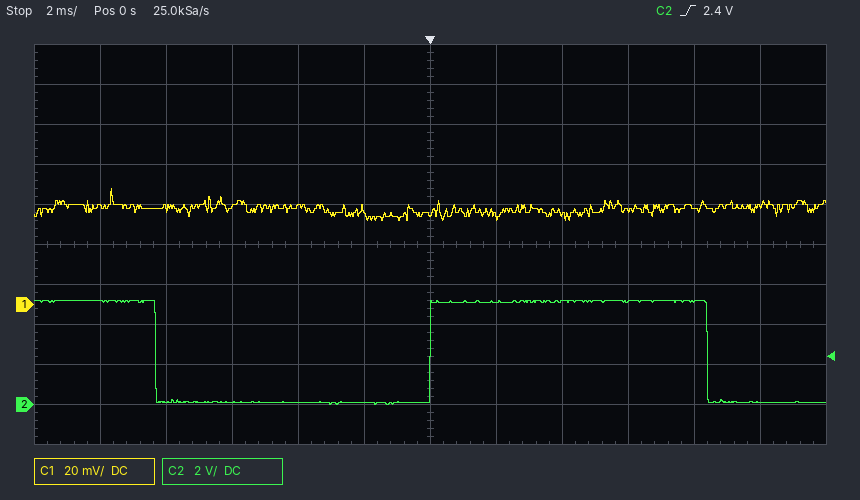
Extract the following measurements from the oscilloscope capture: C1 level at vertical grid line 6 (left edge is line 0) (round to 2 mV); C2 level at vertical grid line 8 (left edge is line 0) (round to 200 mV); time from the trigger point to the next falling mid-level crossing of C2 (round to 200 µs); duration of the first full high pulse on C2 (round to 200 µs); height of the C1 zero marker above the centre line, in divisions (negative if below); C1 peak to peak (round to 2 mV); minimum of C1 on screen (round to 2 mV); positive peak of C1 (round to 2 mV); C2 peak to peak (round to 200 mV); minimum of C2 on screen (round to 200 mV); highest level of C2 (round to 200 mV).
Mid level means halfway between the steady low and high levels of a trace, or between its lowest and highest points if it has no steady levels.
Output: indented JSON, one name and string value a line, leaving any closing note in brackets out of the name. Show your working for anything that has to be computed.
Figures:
{
  "C1 level at vertical grid line 6 (left edge is line 0)": "46 mV",
  "C2 level at vertical grid line 8 (left edge is line 0)": "5.2 V",
  "time from the trigger point to the next falling mid-level crossing of C2": "8.4 ms",
  "duration of the first full high pulse on C2": "8.4 ms",
  "height of the C1 zero marker above the centre line, in divisions": "-1.5 div",
  "C1 peak to peak": "58 mV − (42 mV) = 16 mV",
  "minimum of C1 on screen": "42 mV",
  "positive peak of C1": "58 mV",
  "C2 peak to peak": "5.2 V − (0.0 V) = 5.2 V",
  "minimum of C2 on screen": "0.0 V",
  "highest level of C2": "5.2 V"
}
